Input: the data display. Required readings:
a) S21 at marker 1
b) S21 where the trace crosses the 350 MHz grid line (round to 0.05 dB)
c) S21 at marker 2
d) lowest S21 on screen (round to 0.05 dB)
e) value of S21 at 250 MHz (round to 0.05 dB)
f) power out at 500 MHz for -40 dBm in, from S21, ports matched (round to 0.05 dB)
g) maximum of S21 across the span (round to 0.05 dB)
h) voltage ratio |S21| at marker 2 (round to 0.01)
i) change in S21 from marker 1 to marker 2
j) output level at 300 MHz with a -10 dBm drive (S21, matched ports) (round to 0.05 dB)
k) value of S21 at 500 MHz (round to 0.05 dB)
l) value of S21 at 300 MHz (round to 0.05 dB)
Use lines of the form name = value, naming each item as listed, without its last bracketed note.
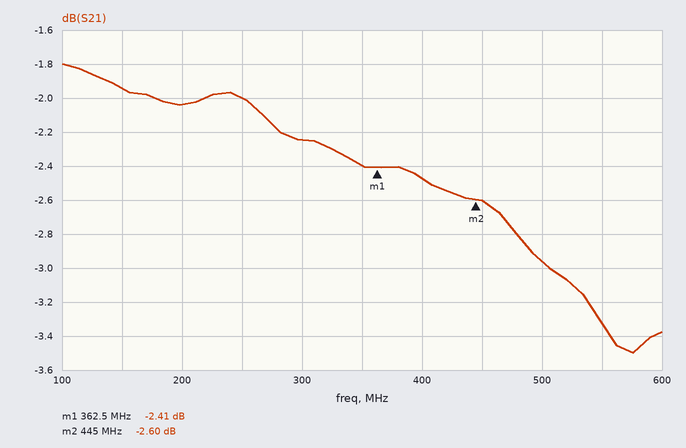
S21 at marker 1 = -2.41 dB
S21 where the trace crosses the 350 MHz grid line = -2.40 dB
S21 at marker 2 = -2.60 dB
lowest S21 on screen = -3.50 dB
value of S21 at 250 MHz = -2.00 dB
power out at 500 MHz for -40 dBm in, from S21, ports matched = -42.95 dBm
maximum of S21 across the span = -1.80 dB
voltage ratio |S21| at marker 2 = 0.74
change in S21 from marker 1 to marker 2 = -0.19 dB
output level at 300 MHz with a -10 dBm drive (S21, matched ports) = -12.25 dBm
value of S21 at 500 MHz = -2.95 dB
value of S21 at 300 MHz = -2.25 dB
